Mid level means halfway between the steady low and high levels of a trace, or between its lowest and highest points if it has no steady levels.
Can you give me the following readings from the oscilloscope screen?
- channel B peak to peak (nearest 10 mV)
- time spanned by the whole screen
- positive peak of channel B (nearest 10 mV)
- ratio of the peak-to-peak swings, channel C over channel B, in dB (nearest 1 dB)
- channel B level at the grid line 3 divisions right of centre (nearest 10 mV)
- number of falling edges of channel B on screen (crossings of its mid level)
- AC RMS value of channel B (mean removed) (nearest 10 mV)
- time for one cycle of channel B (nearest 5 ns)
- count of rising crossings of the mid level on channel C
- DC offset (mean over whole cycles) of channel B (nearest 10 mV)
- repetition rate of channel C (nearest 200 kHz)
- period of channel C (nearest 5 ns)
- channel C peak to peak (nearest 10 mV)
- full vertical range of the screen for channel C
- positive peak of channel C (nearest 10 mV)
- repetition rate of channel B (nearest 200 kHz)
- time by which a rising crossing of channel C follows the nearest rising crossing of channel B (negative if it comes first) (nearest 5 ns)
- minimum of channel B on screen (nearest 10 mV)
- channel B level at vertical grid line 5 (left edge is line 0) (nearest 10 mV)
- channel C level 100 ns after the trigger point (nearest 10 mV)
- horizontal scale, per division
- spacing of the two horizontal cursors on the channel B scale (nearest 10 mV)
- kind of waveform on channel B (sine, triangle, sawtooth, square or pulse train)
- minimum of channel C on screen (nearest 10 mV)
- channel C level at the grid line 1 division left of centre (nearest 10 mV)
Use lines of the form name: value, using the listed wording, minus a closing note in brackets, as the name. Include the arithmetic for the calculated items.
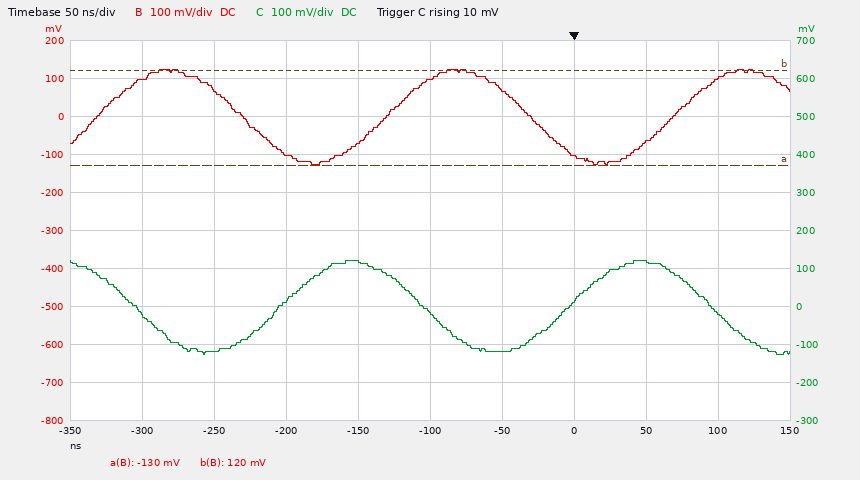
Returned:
channel B peak to peak: 120 mV − (-130 mV) = 250 mV
time spanned by the whole screen: 500 ns
positive peak of channel B: 120 mV
ratio of the peak-to-peak swings, channel C over channel B, in dB: 20 log10(250 mV / 250 mV) ≈ 0 dB
channel B level at the grid line 3 divisions right of centre: -70 mV
number of falling edges of channel B on screen: 2
AC RMS value of channel B (mean removed): 250 mV / (2√2) ≈ 88.4 mV, so 90 mV to the nearest 10 mV
time for one cycle of channel B: 200 ns
count of rising crossings of the mid level on channel C: 2
DC offset (mean over whole cycles) of channel B: (120 mV + (-130 mV)) / 2 ≈ 0 mV
repetition rate of channel C: 1 / 200 ns ≈ 5.0 MHz
period of channel C: 200 ns
channel C peak to peak: 120 mV − (-130 mV) = 250 mV
full vertical range of the screen for channel C: 1 V
positive peak of channel C: 120 mV
repetition rate of channel B: 1 / 200 ns ≈ 5.0 MHz
time by which a rising crossing of channel C follows the nearest rising crossing of channel B (negative if it comes first): -75 ns
minimum of channel B on screen: -130 mV
channel B level at vertical grid line 5 (left edge is line 0): 100 mV
channel C level 100 ns after the trigger point: -20 mV
horizontal scale, per division: 50 ns
spacing of the two horizontal cursors on the channel B scale: 250 mV
kind of waveform on channel B: sine
minimum of channel C on screen: -130 mV
channel C level at the grid line 1 division left of centre: 120 mV
